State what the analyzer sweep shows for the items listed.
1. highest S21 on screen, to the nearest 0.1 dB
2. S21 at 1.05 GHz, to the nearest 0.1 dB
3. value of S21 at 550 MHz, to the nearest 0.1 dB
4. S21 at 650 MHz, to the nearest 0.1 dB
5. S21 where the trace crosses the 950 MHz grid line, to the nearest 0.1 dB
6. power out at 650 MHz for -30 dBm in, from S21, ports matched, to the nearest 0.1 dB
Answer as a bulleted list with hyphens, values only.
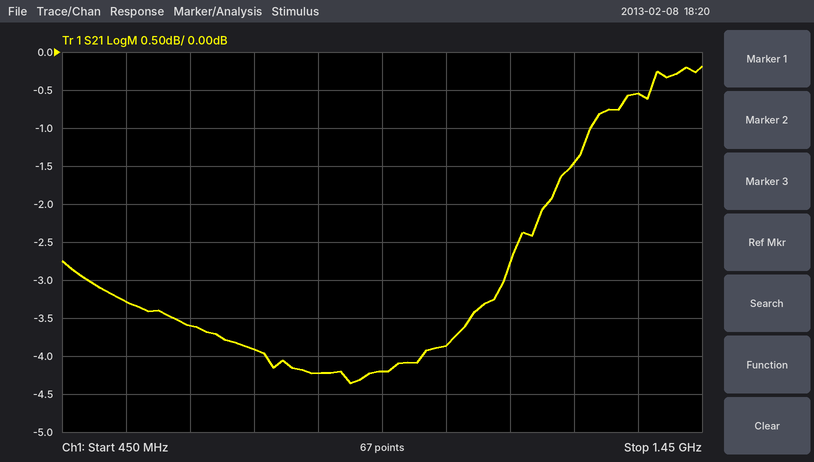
- -0.2 dB
- -3.9 dB
- -3.3 dB
- -3.6 dB
- -4.2 dB
- -33.6 dBm
